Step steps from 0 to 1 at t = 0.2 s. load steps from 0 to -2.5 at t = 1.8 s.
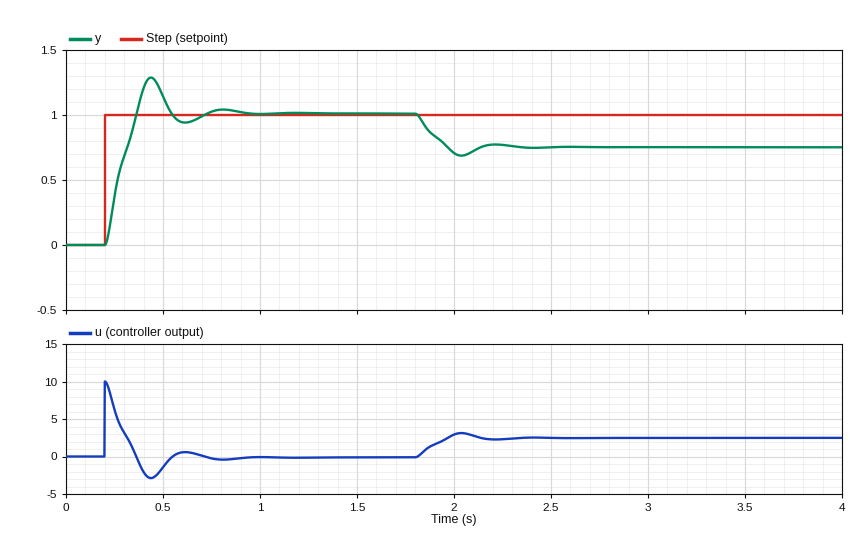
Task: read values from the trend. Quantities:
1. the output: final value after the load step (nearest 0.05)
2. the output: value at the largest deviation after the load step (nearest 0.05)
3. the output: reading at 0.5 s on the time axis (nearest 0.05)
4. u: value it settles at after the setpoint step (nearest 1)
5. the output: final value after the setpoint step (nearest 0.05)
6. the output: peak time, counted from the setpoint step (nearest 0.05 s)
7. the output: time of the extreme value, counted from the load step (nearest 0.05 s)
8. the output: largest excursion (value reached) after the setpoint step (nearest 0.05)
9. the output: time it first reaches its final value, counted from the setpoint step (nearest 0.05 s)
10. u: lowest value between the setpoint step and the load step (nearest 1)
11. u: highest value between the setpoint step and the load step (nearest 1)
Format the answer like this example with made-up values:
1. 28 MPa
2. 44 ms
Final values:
1. 0.75
2. 0.70
3. 1.15
4. 0
5. 1.00
6. 0.25 s
7. 0.25 s
8. 1.30
9. 0.15 s
10. -3
11. 10
